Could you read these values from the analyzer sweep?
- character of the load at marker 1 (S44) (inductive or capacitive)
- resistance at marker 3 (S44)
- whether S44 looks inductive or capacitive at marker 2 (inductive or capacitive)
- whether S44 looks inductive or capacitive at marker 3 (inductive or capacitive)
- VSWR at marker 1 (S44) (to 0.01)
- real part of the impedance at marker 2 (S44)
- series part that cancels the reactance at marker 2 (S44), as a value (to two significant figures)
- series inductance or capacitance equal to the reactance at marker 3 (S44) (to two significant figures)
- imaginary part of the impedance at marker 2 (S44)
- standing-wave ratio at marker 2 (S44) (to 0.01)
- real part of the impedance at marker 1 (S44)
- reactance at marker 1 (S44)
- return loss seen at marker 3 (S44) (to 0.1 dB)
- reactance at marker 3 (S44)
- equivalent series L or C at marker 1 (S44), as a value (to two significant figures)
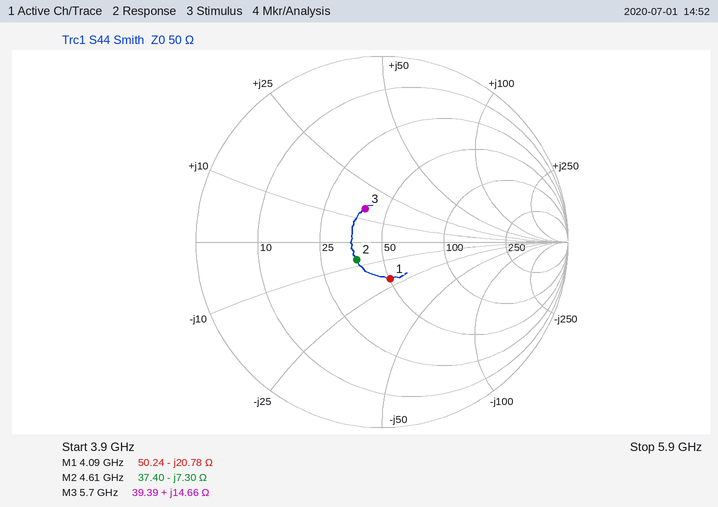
capacitive
39.39 Ω
capacitive
inductive
1.51
37.40 Ω
250 pH
410 pH
-7.30 Ω
1.40
50.24 Ω
-20.78 Ω
14.0 dB
+14.66 Ω
1.9 pF
